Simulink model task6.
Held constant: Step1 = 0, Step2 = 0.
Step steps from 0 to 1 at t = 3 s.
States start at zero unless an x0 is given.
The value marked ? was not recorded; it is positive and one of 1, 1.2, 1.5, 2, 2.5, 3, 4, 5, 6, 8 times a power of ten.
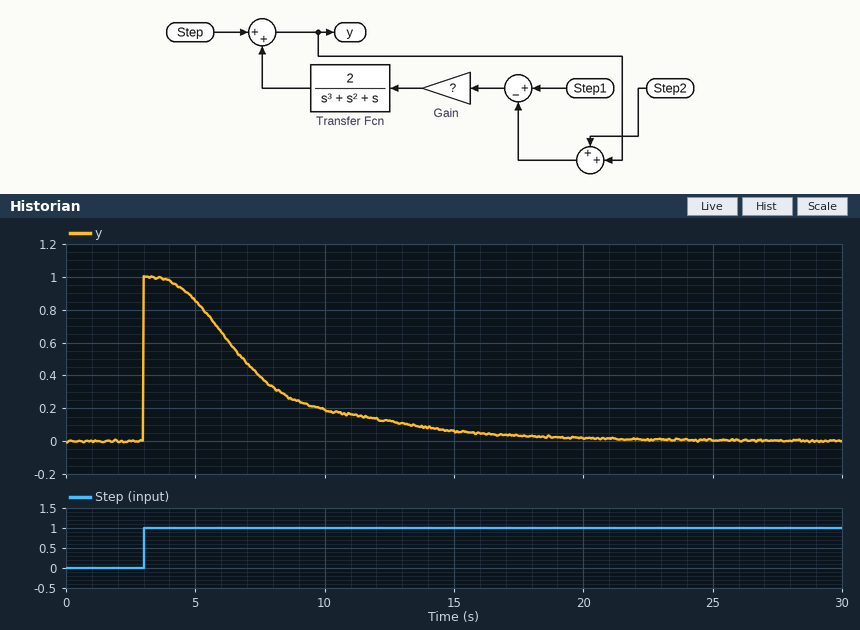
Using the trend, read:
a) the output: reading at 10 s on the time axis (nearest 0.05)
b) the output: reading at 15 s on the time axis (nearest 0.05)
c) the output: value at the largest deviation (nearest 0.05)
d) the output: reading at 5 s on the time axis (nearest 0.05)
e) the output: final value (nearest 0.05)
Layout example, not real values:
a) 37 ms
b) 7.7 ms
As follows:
a) 0.20
b) 0.05
c) 1.00
d) 0.85
e) 0.00
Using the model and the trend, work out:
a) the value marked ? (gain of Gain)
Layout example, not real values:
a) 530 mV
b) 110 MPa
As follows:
a) 0.1
